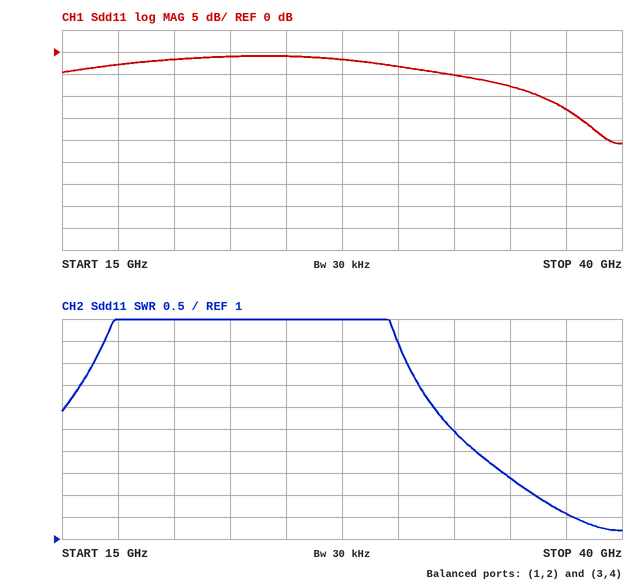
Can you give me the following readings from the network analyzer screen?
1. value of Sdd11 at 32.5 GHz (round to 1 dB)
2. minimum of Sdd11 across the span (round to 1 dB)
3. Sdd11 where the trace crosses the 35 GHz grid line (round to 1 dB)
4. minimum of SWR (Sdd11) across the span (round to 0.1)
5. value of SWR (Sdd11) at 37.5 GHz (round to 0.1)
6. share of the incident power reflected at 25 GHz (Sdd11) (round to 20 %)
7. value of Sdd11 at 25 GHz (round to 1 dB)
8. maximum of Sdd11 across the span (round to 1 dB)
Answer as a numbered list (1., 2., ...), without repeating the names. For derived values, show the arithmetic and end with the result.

1. -5 dB
2. -21 dB
3. -8 dB
4. 1.2
5. 1.6
6. 10^(-1/10) ≈ 79.4 %, so 80 % to the nearest 20 %
7. -1 dB
8. -1 dB
